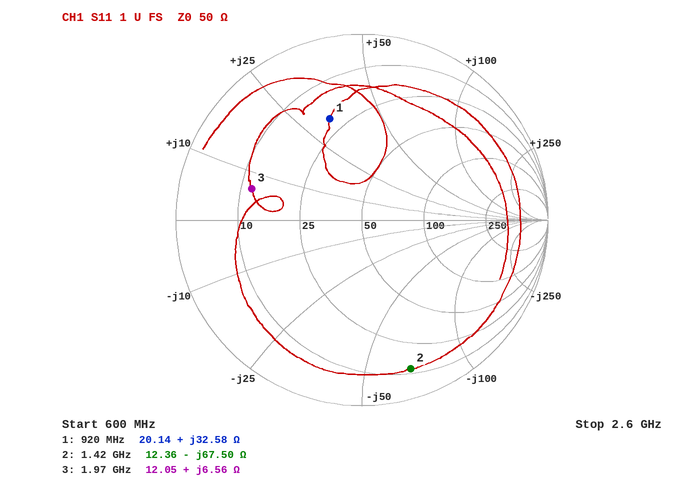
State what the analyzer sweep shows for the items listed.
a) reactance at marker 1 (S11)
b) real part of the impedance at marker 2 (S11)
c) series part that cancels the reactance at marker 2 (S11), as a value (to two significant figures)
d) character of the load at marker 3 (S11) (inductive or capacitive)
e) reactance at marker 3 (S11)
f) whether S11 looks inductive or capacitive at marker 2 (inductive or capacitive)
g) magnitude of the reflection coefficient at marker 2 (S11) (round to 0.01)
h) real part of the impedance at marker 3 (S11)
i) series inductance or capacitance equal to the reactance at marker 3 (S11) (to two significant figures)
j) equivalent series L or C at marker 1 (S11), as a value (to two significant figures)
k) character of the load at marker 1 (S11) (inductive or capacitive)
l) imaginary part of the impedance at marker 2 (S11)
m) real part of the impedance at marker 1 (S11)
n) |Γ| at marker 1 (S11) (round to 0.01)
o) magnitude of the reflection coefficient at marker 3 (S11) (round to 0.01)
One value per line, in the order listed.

+32.58 Ω
12.36 Ω
7.6 nH
inductive
+6.56 Ω
capacitive
0.84
12.05 Ω
530 pH
5.6 nH
inductive
-67.50 Ω
20.14 Ω
0.57
0.62
